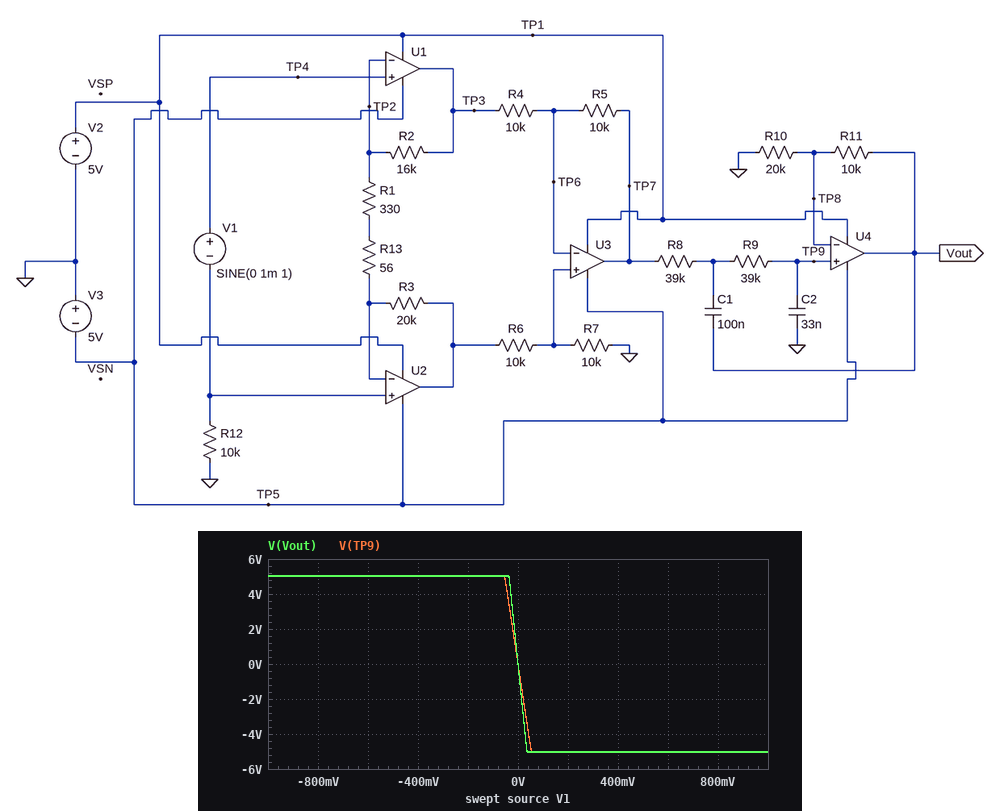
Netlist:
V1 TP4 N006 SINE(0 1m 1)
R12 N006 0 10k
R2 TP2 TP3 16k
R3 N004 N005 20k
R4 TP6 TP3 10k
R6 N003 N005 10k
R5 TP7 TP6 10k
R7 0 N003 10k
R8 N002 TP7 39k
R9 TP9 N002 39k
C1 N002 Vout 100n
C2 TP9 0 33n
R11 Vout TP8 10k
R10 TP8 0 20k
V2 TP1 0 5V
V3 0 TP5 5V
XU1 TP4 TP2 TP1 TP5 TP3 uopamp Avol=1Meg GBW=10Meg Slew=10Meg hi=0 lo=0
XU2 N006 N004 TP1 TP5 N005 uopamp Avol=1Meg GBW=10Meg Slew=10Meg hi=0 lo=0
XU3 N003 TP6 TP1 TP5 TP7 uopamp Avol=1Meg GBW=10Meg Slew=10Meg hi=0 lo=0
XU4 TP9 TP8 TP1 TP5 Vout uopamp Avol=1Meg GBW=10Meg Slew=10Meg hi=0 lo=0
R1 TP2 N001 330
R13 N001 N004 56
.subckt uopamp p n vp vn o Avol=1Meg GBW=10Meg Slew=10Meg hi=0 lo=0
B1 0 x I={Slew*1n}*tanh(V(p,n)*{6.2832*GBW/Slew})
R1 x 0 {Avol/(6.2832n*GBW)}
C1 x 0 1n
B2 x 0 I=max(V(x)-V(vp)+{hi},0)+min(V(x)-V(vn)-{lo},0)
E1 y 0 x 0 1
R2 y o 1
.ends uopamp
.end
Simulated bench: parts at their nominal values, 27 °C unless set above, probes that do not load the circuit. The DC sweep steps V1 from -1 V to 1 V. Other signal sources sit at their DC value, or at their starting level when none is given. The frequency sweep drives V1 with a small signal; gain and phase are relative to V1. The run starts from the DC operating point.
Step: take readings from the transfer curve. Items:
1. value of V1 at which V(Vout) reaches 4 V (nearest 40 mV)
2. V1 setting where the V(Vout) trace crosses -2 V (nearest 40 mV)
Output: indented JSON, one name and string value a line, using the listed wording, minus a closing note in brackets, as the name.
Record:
{
  "value of V1 at which V(Vout) reaches 4 V": "-40 mV",
  "V1 setting where the V(Vout) trace crosses -2 V": "0 V"
}
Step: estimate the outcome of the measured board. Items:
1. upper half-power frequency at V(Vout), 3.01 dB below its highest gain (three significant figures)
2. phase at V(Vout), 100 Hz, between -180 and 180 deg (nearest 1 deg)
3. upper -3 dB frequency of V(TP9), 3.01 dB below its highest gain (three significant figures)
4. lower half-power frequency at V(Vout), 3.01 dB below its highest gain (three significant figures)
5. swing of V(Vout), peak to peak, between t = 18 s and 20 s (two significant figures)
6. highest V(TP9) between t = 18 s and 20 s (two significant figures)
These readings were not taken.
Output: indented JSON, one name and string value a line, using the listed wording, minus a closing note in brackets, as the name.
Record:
{
  "upper half-power frequency at V(Vout), 3.01 dB below its highest gain": "79.0 Hz",
  "phase at V(Vout), 100 Hz, between -180 and 180 deg": "22 deg",
  "upper -3 dB frequency of V(TP9), 3.01 dB below its highest gain": "79.0 Hz",
  "lower half-power frequency at V(Vout), 3.01 dB below its highest gain": "58.8 Hz",
  "swing of V(Vout), peak to peak, between t = 18 s and 20 s": "280 mV",
  "highest V(TP9) between t = 18 s and 20 s": "94 mV"
}
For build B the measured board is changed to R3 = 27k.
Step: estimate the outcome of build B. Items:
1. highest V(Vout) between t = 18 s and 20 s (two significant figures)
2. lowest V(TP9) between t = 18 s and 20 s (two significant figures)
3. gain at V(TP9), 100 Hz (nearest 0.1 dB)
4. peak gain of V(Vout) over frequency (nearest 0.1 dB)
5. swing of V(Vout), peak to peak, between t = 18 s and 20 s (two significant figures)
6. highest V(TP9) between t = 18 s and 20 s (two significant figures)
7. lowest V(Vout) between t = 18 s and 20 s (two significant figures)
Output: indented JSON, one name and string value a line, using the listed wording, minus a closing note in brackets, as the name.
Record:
{
  "highest V(Vout) between t = 18 s and 20 s": "170 mV",
  "lowest V(TP9) between t = 18 s and 20 s": "-110 mV",
  "gain at V(TP9), 100 Hz": "40.5 dB",
  "peak gain of V(Vout) over frequency": "55.7 dB",
  "swing of V(Vout), peak to peak, between t = 18 s and 20 s": "340 mV",
  "highest V(TP9) between t = 18 s and 20 s": "110 mV",
  "lowest V(Vout) between t = 18 s and 20 s": "-170 mV"
}
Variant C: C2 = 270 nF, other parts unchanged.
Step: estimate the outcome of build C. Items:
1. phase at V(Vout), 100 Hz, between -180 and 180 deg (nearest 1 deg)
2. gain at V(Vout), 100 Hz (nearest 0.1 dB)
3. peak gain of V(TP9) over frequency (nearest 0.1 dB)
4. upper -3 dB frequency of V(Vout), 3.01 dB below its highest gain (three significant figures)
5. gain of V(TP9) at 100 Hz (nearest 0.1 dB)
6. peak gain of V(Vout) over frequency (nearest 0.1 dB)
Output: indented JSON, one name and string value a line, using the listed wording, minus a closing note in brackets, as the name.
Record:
{
  "phase at V(Vout), 100 Hz, between -180 and 180 deg": "38 deg",
  "gain at V(Vout), 100 Hz": "17.3 dB",
  "peak gain of V(TP9) over frequency": "39.5 dB",
  "upper -3 dB frequency of V(Vout), 3.01 dB below its highest gain": "9.36 Hz",
  "gain of V(TP9) at 100 Hz": "13.7 dB",
  "peak gain of V(Vout) over frequency": "43.0 dB"
}
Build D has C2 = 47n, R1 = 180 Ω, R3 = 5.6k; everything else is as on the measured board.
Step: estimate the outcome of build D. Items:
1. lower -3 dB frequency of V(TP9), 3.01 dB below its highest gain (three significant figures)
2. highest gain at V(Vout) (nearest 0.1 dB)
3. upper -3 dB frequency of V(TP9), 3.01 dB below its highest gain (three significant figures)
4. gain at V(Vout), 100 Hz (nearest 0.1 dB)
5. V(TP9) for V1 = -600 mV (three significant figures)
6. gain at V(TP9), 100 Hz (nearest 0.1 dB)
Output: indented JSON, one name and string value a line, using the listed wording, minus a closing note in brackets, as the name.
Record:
{
  "lower -3 dB frequency of V(TP9), 3.01 dB below its highest gain": "25.7 Hz",
  "highest gain at V(Vout)": "47.2 dB",
  "upper -3 dB frequency of V(TP9), 3.01 dB below its highest gain": "70.5 Hz",
  "gain at V(Vout), 100 Hz": "36.3 dB",
  "V(TP9) for V1 = -600 mV": "5.01 V",
  "gain at V(TP9), 100 Hz": "32.8 dB"
}
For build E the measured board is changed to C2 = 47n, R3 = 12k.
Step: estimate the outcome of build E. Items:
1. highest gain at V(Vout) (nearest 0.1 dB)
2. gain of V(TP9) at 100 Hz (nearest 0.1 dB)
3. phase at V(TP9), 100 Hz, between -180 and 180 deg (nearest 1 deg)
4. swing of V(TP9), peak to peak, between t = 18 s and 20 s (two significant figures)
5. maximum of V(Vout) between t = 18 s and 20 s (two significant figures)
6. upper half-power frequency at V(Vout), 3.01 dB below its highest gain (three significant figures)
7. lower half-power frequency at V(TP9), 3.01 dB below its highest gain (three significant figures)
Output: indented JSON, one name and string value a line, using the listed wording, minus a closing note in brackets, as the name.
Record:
{
  "highest gain at V(Vout)": "45.2 dB",
  "gain of V(TP9) at 100 Hz": "30.8 dB",
  "phase at V(TP9), 100 Hz, between -180 and 180 deg": "31 deg",
  "swing of V(TP9), peak to peak, between t = 18 s and 20 s": "150 mV",
  "maximum of V(Vout) between t = 18 s and 20 s": "110 mV",
  "upper half-power frequency at V(Vout), 3.01 dB below its highest gain": "70.5 Hz",
  "lower half-power frequency at V(TP9), 3.01 dB below its highest gain": "25.7 Hz"
}
